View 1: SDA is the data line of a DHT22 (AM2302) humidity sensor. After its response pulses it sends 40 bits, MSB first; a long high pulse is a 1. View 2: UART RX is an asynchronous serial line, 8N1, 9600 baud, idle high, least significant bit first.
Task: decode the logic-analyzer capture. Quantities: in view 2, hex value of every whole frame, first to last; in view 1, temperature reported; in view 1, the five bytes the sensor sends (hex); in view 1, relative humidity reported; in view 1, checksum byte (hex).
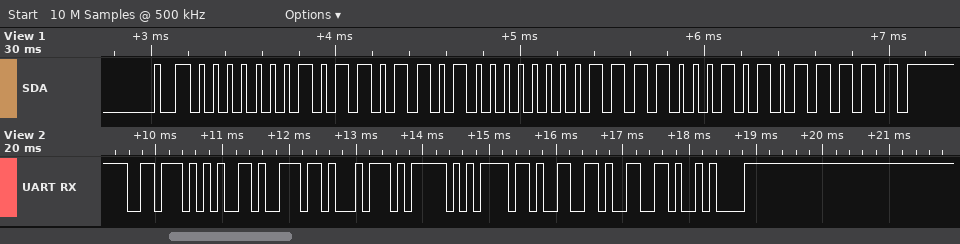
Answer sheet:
0x76 0x65 0x6E 0x74 0x5F 0x6F 0x66 0x66 0x0A
24.1 °C
01 6D 00 F1 5F
36.5 %
0x5F
